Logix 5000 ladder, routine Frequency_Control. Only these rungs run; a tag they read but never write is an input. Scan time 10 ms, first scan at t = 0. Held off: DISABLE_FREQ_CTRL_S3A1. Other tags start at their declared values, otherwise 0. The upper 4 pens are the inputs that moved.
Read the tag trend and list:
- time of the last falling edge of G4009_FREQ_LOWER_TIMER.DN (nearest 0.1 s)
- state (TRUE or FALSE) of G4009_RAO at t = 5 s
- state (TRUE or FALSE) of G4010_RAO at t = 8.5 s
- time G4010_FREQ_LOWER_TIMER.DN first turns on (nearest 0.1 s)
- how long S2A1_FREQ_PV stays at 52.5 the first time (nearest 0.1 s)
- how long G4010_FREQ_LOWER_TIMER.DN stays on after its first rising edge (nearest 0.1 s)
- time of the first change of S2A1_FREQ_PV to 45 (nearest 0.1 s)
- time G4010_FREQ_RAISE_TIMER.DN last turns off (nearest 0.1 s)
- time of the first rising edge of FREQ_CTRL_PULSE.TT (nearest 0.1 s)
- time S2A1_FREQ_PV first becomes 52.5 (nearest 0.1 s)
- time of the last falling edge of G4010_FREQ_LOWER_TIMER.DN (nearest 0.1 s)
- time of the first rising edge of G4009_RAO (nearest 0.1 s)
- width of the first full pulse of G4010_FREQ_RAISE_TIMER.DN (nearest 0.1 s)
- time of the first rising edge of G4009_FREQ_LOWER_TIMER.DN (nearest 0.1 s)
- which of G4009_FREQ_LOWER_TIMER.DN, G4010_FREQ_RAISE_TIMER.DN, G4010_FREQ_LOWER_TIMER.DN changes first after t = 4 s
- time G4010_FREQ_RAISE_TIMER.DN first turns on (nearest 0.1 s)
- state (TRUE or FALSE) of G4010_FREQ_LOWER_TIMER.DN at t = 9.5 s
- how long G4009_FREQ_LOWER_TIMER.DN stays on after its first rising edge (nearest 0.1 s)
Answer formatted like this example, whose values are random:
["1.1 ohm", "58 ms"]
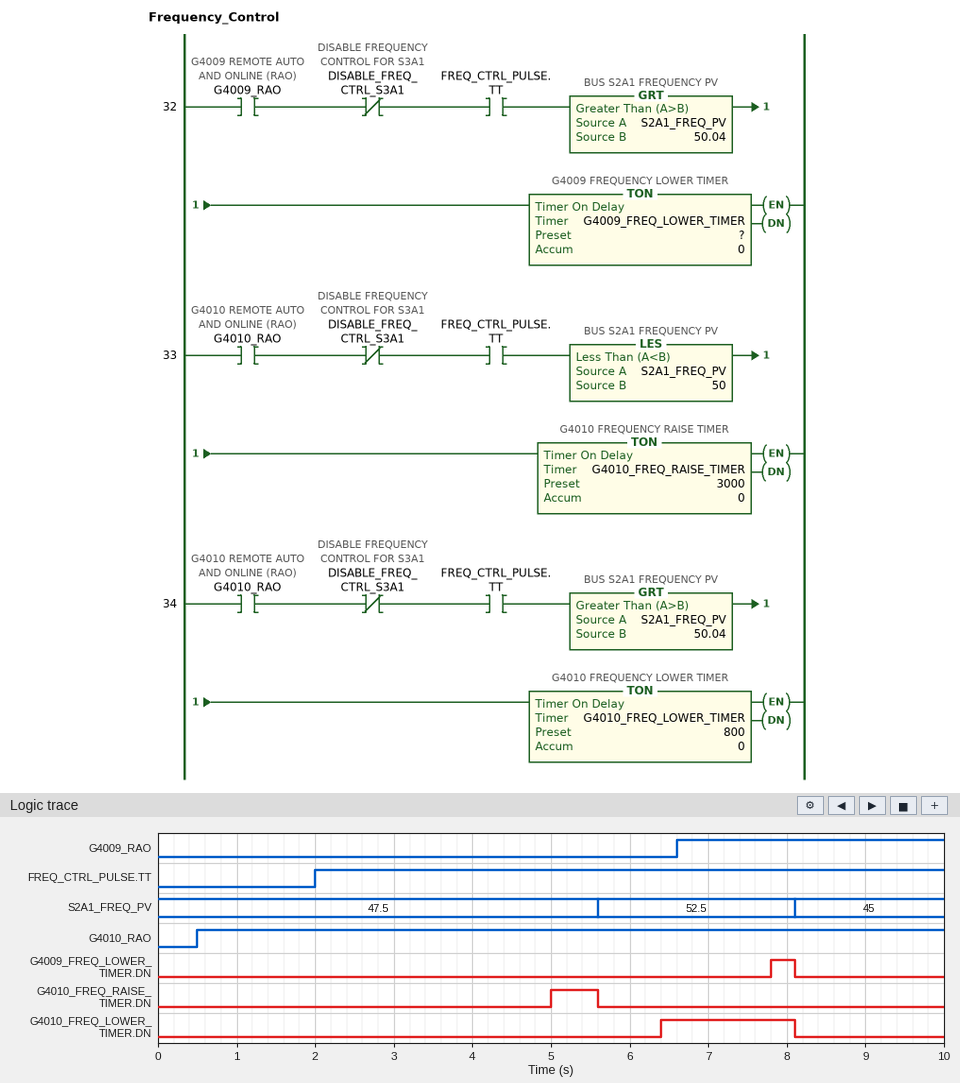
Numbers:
["8.1 s", "FALSE", "TRUE", "6.4 s", "2.5 s", "1.7 s", "8.1 s", "5.6 s", "2.0 s", "5.6 s", "8.1 s", "6.6 s", "0.6 s", "7.8 s", "G4010_FREQ_RAISE_TIMER.DN", "5.0 s", "FALSE", "0.3 s"]
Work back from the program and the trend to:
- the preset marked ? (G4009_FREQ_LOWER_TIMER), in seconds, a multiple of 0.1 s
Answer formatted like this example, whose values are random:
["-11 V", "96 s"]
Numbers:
["1.2 s"]
